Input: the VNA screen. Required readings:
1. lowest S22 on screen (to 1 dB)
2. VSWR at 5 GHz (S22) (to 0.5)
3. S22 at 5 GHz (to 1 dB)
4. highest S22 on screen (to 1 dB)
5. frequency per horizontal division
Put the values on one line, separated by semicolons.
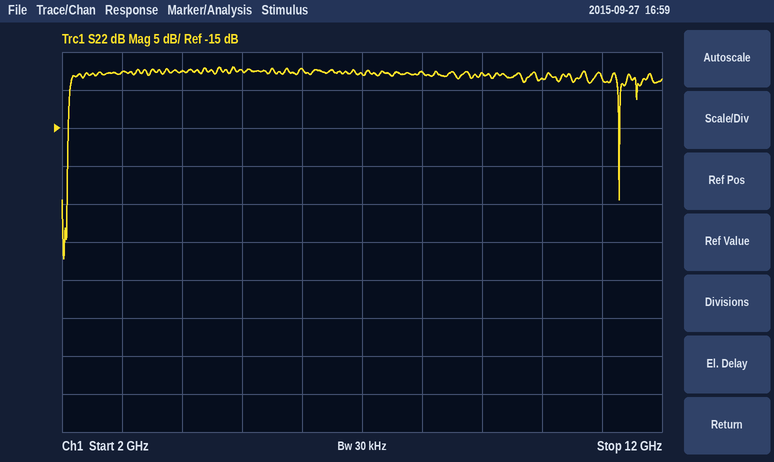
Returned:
-32 dB; 2.5; -7 dB; -7 dB; 1 GHz
